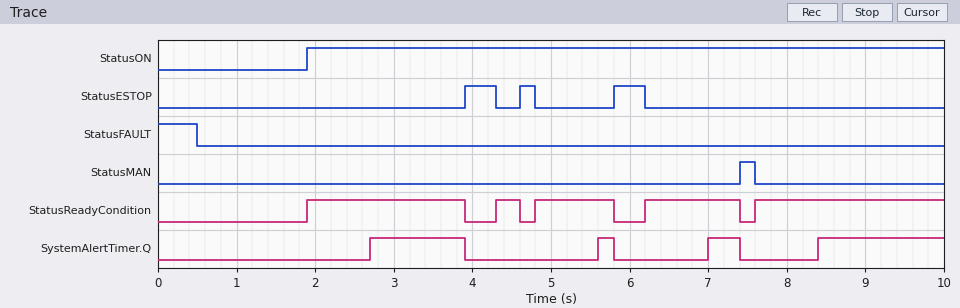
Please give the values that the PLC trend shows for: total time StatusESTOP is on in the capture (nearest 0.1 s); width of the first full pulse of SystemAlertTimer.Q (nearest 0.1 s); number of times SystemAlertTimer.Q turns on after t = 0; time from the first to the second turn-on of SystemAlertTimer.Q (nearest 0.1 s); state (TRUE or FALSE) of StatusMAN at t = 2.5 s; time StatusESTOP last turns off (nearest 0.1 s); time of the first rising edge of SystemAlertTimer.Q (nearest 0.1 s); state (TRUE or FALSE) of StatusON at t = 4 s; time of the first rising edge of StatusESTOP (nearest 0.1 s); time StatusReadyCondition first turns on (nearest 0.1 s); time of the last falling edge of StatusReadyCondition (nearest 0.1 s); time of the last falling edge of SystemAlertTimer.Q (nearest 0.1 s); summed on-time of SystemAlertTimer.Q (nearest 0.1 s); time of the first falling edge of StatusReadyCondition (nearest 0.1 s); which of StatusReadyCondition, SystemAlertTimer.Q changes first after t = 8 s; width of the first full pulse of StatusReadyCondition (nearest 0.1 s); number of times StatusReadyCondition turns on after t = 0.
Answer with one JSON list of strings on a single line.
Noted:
["1.0 s", "1.2 s", "4", "2.9 s", "FALSE", "6.2 s", "2.7 s", "TRUE", "3.9 s", "1.9 s", "7.4 s", "7.4 s", "3.4 s", "3.9 s", "SystemAlertTimer.Q", "2.0 s", "5"]
